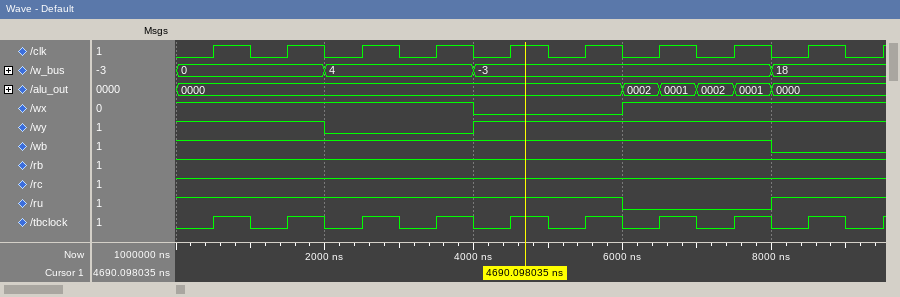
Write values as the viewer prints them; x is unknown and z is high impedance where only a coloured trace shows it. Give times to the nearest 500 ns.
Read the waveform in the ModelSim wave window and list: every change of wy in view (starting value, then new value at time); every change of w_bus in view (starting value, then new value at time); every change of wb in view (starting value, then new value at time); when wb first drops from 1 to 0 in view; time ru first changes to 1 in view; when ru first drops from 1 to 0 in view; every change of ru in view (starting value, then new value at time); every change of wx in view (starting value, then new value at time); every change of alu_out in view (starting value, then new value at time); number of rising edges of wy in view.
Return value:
1, 0 at 2000 ns, 1 at 4000 ns
0, 4 at 2000 ns, -3 at 4000 ns, 18 at 8000 ns
1, 0 at 8000 ns
8000 ns
8000 ns
6000 ns
1, 0 at 6000 ns, 1 at 8000 ns
1, 0 at 4000 ns, 1 at 6000 ns
0000, 0002 at 6000 ns, 0001 at 6500 ns, 0002 at 7000 ns, 0001 at 7500 ns, 0000 at 8000 ns
1
